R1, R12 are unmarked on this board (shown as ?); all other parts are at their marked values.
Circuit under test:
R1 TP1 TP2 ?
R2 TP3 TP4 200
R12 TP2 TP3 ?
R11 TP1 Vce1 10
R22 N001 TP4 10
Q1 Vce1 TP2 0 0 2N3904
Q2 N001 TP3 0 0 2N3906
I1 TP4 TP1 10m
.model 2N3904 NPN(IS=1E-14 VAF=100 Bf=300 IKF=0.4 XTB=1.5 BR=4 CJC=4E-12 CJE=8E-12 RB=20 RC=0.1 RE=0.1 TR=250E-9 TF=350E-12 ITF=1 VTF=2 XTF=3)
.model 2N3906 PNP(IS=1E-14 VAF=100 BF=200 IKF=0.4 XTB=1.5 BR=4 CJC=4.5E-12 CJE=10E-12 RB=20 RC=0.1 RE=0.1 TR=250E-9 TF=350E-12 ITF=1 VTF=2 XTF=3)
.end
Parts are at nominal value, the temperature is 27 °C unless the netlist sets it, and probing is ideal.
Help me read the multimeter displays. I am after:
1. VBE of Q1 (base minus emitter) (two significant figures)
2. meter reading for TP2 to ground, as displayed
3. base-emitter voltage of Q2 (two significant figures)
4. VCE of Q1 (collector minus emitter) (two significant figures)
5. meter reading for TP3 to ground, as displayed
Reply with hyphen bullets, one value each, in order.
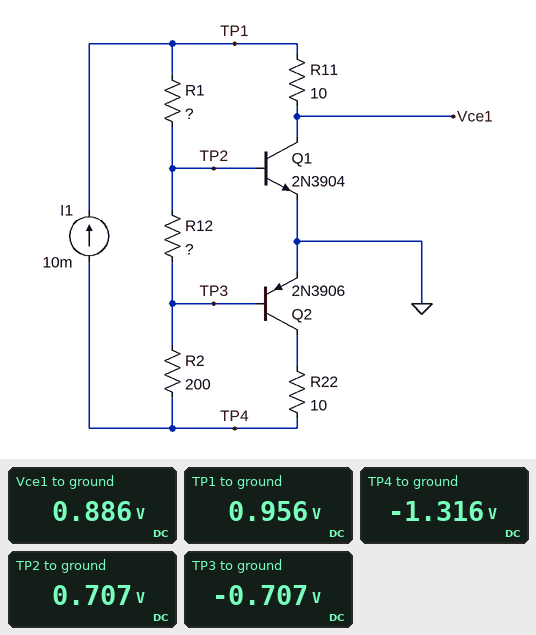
- 710 mV
- 0.707 V
- -710 mV
- 890 mV
- -0.707 V
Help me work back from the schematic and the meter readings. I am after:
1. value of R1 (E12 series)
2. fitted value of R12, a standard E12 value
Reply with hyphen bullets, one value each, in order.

- 82 Ω
- 470 Ω
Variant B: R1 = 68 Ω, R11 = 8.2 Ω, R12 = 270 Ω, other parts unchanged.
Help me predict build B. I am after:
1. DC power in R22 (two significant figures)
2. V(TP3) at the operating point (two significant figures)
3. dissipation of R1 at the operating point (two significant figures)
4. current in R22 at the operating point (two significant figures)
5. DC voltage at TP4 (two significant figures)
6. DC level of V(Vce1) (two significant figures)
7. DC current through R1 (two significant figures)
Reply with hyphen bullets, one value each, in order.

- 230 µW
- -700 mV
- 1.8 mW
- 4.8 mA
- -1.7 V
- 1.0 V
- 5.2 mA
